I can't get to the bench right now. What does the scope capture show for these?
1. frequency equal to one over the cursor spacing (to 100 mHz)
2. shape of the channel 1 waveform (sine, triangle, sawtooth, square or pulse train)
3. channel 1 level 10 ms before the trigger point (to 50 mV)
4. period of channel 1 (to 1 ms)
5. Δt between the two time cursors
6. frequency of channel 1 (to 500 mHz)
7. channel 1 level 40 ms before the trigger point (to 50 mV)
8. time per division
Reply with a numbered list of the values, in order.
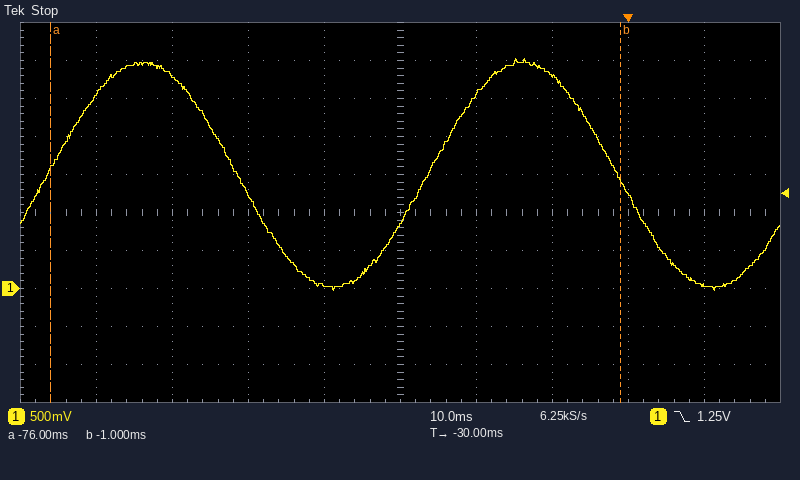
1. 13.3 Hz
2. sine
3. 2.80 V
4. 50 ms
5. 75 ms
6. 20.0 Hz
7. 50 mV
8. 10 ms
